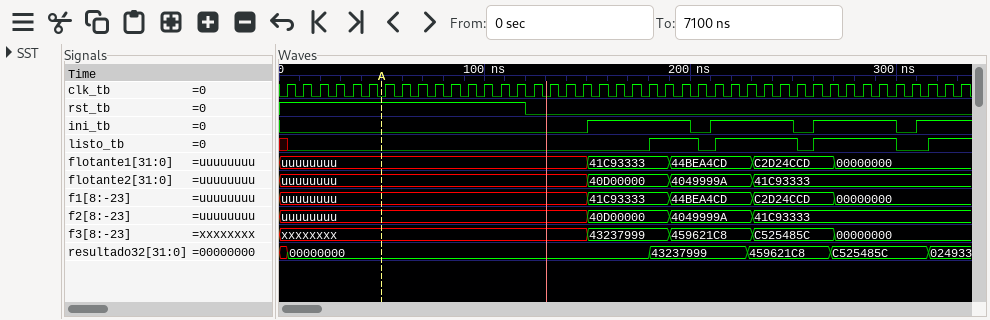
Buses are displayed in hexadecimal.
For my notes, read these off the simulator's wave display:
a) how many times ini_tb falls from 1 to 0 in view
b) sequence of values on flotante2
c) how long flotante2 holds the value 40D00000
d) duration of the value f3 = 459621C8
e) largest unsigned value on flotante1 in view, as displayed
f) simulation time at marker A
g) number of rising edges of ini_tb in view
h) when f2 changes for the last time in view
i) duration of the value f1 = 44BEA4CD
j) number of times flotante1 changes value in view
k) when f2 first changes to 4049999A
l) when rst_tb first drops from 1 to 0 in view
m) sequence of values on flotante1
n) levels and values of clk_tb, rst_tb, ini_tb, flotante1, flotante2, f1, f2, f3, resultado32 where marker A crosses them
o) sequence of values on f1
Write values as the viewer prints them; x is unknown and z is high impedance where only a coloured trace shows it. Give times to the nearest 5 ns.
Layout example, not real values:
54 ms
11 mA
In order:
3
uuuuuuuu, 40D00000, 4049999A, 41C93333
40 ns
40 ns
C2D24CCD
50 ns
4
230 ns
40 ns
4
190 ns
120 ns
uuuuuuuu, 41C93333, 44BEA4CD, C2D24CCD, 00000000
clk_tb=0, rst_tb=1, ini_tb=0, flotante1=uuuuuuuu, flotante2=uuuuuuuu, f1=uuuuuuuu, f2=uuuuuuuu, f3=xxxxxxxx, resultado32=00000000
uuuuuuuu, 41C93333, 44BEA4CD, C2D24CCD, 00000000
